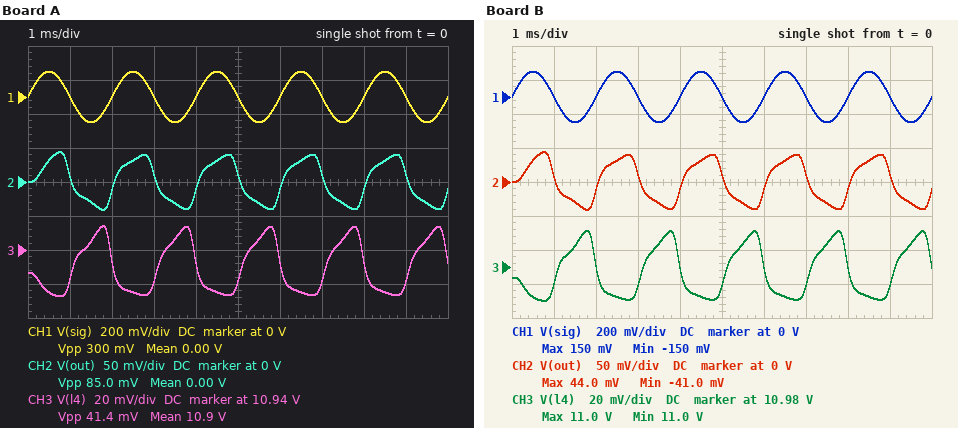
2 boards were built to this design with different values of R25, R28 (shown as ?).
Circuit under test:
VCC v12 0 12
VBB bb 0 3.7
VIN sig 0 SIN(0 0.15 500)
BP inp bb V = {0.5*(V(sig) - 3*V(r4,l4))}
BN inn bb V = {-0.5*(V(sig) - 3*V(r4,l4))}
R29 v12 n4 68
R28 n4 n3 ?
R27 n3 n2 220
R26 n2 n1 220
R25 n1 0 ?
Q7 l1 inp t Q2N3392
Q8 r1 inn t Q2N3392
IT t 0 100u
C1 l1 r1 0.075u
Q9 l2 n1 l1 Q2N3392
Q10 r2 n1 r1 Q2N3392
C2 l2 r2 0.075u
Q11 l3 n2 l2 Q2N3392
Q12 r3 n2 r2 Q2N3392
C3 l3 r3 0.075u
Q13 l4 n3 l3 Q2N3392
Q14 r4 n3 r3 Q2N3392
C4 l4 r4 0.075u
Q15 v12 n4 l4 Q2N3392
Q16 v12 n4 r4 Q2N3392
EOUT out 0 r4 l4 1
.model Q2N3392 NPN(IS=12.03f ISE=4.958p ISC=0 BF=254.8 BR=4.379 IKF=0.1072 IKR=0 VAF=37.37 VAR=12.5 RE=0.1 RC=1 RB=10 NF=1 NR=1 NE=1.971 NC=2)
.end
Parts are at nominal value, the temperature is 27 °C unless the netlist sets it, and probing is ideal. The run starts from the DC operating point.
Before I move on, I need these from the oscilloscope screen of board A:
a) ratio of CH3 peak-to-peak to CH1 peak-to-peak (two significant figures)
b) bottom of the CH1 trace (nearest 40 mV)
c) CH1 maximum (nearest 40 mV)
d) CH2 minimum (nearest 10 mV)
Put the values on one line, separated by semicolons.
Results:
0.14; -160 mV; 160 mV; -40 mV
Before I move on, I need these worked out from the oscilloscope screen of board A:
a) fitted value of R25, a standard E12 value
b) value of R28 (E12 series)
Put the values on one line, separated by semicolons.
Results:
560 Ω; 560 Ω
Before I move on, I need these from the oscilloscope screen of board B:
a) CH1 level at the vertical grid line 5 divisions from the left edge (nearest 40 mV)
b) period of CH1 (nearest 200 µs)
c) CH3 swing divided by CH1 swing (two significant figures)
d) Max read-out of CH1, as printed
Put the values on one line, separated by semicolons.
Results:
0 V; 2.0 ms; 0.14; 150 mV
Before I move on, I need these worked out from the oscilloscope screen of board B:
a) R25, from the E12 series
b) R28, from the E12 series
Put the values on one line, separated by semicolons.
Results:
820 Ω; 470 Ω
